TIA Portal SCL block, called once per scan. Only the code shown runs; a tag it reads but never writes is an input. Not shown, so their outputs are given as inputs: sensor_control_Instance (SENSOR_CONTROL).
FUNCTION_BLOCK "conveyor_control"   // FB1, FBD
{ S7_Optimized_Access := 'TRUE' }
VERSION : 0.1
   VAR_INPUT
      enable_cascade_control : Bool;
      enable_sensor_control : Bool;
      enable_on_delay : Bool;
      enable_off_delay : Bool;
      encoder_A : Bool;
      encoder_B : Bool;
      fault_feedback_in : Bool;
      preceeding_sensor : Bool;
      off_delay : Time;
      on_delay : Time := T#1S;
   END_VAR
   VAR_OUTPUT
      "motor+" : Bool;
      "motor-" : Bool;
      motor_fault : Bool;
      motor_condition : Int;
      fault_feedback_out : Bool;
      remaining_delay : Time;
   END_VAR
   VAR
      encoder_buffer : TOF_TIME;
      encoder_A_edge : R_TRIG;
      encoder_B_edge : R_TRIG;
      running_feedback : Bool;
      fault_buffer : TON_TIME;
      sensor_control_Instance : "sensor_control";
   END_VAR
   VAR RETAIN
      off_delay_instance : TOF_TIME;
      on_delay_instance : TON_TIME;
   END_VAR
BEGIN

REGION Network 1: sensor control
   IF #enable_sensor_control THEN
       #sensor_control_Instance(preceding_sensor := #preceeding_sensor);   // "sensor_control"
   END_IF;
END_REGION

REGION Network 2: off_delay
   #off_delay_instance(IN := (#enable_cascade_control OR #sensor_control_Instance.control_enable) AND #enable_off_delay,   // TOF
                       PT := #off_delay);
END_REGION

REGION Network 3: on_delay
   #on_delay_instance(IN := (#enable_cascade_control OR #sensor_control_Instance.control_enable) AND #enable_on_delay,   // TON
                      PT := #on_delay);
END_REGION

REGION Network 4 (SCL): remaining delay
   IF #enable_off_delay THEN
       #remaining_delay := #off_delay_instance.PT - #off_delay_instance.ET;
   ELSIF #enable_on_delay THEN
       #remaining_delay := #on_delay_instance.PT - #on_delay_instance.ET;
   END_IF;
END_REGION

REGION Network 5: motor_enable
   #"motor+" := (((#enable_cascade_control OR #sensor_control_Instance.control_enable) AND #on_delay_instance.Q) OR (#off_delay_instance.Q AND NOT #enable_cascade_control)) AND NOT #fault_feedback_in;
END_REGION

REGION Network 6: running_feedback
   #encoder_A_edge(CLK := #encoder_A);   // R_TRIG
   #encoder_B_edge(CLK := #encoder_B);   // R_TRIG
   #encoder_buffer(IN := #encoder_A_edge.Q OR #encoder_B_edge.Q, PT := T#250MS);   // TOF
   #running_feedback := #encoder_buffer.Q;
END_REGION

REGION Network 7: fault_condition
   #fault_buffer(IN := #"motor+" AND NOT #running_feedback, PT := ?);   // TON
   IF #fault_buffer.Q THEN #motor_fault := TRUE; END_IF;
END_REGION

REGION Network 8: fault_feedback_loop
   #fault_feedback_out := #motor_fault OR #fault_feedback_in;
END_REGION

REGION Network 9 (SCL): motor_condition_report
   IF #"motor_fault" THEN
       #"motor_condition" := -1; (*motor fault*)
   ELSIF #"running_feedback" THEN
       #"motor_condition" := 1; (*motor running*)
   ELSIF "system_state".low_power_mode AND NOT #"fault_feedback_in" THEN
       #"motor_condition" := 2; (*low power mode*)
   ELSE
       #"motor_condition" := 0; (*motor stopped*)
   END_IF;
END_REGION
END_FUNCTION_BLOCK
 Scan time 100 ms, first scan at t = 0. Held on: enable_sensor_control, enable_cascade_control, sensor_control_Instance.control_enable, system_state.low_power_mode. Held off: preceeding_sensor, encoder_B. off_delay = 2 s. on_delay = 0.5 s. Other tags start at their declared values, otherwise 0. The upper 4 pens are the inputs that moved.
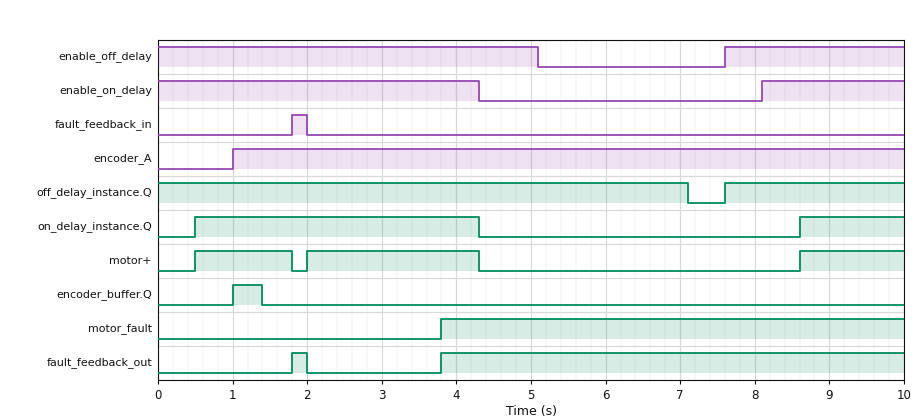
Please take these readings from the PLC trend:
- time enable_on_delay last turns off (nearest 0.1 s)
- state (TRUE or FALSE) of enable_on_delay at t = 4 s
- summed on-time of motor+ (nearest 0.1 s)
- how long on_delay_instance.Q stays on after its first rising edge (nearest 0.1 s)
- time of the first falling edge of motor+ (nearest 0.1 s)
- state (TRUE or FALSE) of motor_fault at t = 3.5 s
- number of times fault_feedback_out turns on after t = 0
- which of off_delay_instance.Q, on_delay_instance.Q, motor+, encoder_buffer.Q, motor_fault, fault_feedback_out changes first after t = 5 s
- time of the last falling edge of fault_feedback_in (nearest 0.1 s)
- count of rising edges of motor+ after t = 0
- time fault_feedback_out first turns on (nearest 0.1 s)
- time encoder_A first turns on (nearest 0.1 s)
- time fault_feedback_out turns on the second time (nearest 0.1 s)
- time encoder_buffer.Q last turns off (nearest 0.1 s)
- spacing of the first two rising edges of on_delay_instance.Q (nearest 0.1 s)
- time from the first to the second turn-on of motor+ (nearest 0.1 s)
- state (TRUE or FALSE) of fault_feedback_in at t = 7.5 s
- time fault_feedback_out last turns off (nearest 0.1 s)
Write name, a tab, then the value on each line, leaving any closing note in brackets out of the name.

time enable_on_delay last turns off	4.3 s
state (TRUE or FALSE) of enable_on_delay at t = 4 s	TRUE
summed on-time of motor+	5.0 s
how long on_delay_instance.Q stays on after its first rising edge	3.8 s
time of the first falling edge of motor+	1.8 s
state (TRUE or FALSE) of motor_fault at t = 3.5 s	FALSE
number of times fault_feedback_out turns on after t = 0	2
which of off_delay_instance.Q, on_delay_instance.Q, motor+, encoder_buffer.Q, motor_fault, fault_feedback_out changes first after t = 5 s	off_delay_instance.Q
time of the last falling edge of fault_feedback_in	2.0 s
count of rising edges of motor+ after t = 0	3
time fault_feedback_out first turns on	1.8 s
time encoder_A first turns on	1.0 s
time fault_feedback_out turns on the second time	3.8 s
time encoder_buffer.Q last turns off	1.4 s
spacing of the first two rising edges of on_delay_instance.Q	8.1 s
time from the first to the second turn-on of motor+	1.5 s
state (TRUE or FALSE) of fault_feedback_in at t = 7.5 s	FALSE
time fault_feedback_out last turns off	2.0 s
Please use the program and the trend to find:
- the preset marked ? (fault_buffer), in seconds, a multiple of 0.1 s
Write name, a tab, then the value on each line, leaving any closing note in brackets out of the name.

the preset marked ? (fault_buffer), in seconds, a multiple of 0.1 s	1.8 s
